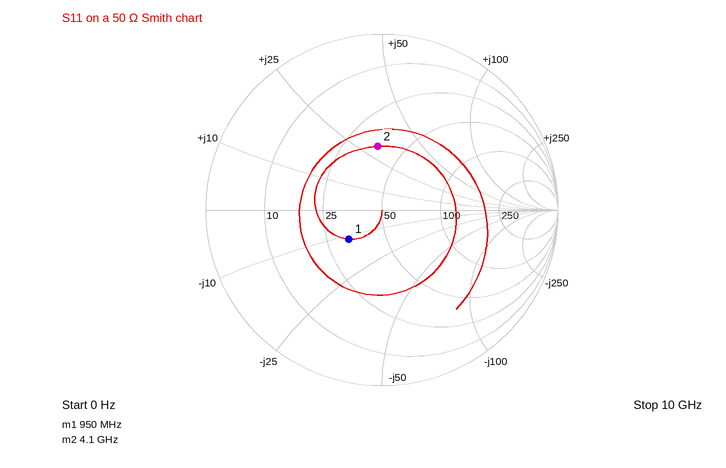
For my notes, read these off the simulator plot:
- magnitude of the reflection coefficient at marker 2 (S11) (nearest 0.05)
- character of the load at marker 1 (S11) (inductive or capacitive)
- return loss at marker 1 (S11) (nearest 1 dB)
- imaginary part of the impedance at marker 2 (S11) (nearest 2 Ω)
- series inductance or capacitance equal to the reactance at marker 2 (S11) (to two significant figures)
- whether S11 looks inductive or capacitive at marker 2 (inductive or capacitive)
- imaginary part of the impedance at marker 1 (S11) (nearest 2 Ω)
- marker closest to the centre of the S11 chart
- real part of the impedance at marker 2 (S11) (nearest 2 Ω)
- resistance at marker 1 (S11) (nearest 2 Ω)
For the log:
0.35
capacitive
12 dB
+30 Ω
1.2 nH
inductive
-12 Ω
marker 1
36 Ω
32 Ω
